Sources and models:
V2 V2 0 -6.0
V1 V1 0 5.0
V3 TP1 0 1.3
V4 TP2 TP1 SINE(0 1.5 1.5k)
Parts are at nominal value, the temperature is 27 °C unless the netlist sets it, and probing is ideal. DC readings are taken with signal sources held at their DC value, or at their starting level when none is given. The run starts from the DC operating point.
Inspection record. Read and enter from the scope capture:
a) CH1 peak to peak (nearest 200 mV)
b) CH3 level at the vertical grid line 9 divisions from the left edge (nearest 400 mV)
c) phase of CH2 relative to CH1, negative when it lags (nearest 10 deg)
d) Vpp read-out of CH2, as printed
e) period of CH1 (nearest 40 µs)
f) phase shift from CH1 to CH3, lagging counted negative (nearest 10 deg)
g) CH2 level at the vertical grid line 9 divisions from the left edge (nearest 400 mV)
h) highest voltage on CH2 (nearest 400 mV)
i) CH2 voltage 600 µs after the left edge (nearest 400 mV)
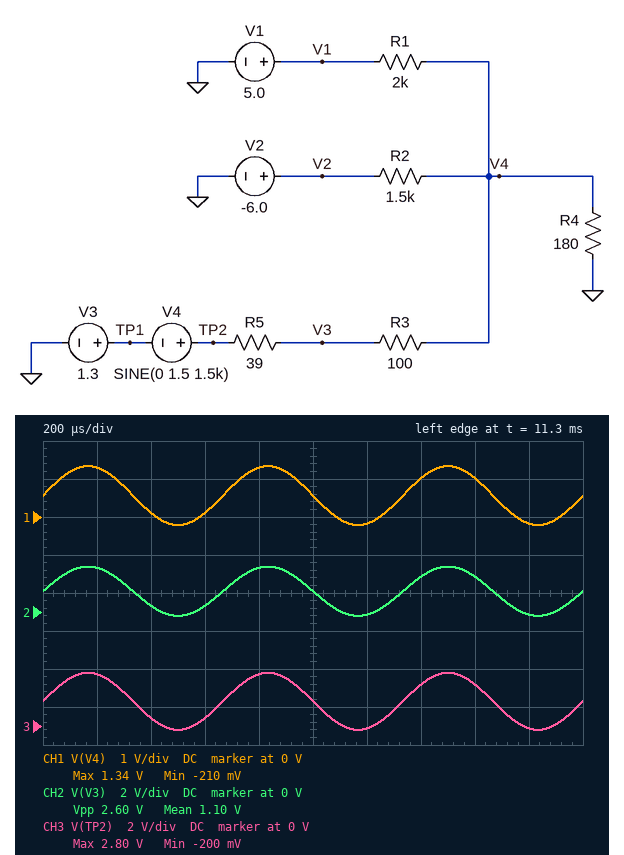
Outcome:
1.6 V
0 V
0 deg
2.60 V
680 µs
0 deg
0 V
2.4 V
400 mV
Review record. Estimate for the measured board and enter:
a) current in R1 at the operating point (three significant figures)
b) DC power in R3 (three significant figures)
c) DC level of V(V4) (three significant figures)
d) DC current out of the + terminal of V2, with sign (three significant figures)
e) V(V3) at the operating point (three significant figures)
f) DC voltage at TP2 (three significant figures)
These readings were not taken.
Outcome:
2.22 mA
2.80 mW
564 mV
-4.38 mA
1.09 V
1.30 V
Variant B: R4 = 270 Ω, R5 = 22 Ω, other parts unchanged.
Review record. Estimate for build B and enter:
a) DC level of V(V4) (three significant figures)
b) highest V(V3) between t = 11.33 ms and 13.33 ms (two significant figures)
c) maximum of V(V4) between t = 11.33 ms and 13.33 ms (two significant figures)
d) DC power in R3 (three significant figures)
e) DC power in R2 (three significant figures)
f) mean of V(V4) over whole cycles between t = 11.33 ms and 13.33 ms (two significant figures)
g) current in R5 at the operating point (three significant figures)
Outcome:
701 mV
2.6 V
1.6 V
2.41 mW
29.9 mW
700 mV
4.91 mA
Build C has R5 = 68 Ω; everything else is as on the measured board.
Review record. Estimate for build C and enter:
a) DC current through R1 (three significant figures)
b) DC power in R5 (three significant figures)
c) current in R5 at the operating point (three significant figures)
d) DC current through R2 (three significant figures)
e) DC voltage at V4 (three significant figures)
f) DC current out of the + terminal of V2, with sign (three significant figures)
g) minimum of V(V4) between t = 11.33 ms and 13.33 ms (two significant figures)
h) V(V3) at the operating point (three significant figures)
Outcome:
2.25 mA
1.57 mW
4.81 mA
4.33 mA
492 mV
-4.33 mA
-210 mV
973 mV
